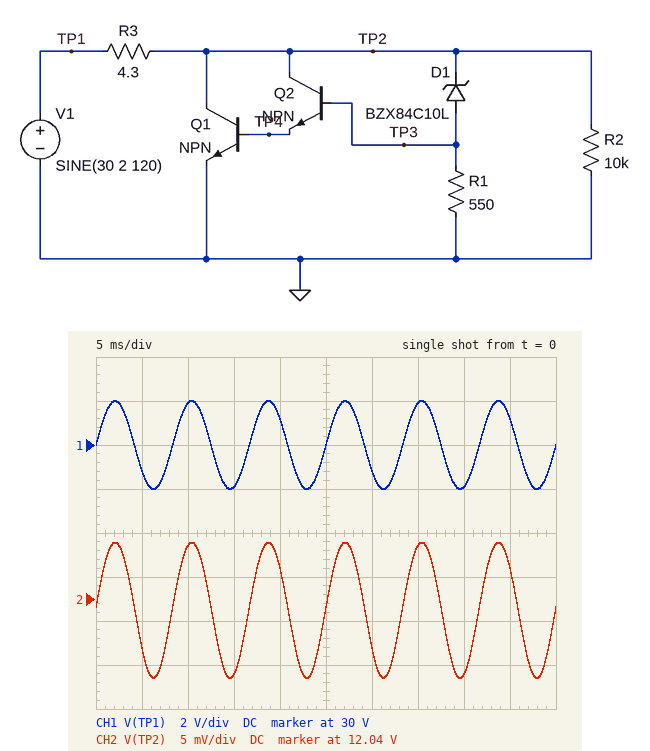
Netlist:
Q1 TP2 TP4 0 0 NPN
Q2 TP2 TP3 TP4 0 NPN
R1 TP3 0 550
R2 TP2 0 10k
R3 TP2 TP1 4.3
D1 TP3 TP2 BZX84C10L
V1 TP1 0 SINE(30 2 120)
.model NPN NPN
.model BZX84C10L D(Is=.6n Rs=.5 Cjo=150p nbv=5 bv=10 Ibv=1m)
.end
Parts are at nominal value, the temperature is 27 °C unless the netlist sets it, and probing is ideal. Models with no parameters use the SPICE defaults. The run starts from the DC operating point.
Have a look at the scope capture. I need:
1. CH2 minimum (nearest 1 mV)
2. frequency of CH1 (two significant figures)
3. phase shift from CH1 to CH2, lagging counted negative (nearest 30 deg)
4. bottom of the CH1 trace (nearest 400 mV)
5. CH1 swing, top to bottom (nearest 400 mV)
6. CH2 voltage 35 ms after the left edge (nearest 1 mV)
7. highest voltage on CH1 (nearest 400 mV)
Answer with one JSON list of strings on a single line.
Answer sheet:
["12.026 V", "120 Hz", "0 deg", "28.0 V", "4.0 V", "12.041 V", "32.0 V"]
